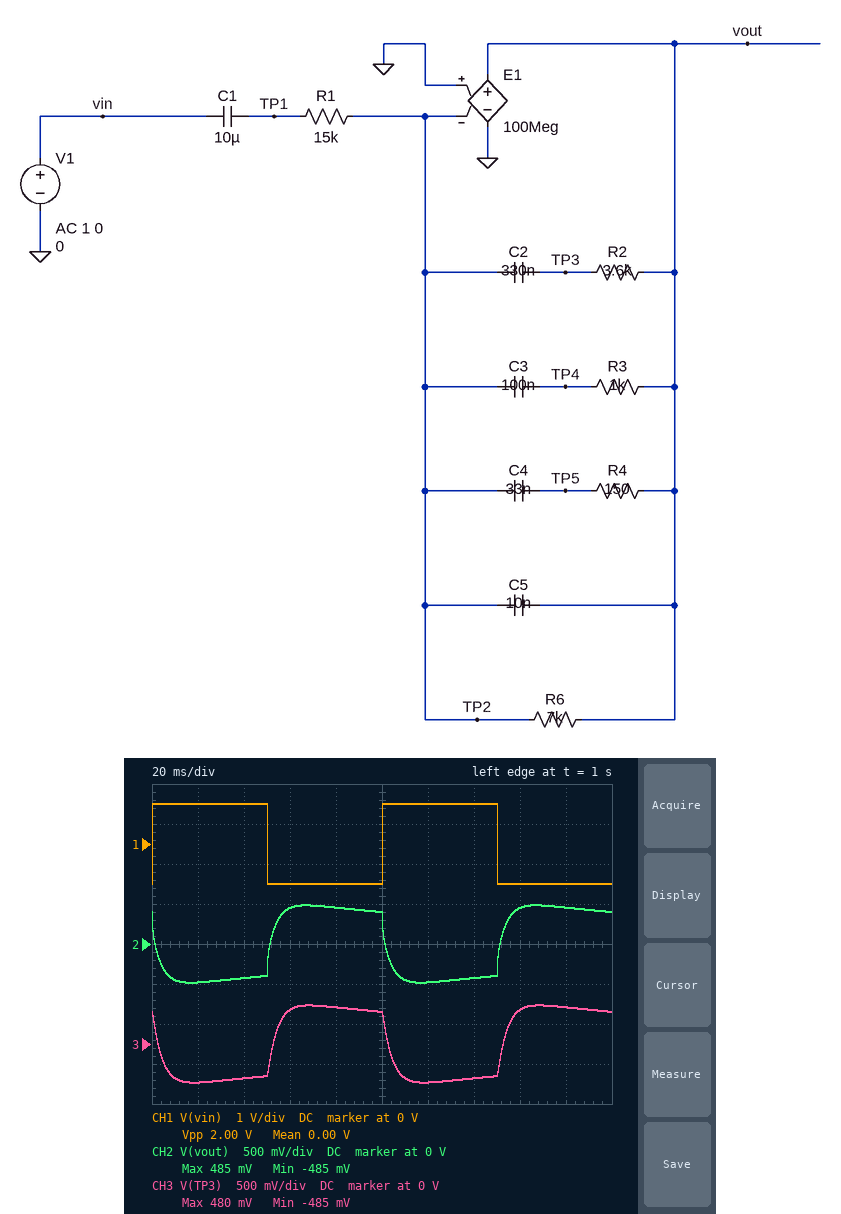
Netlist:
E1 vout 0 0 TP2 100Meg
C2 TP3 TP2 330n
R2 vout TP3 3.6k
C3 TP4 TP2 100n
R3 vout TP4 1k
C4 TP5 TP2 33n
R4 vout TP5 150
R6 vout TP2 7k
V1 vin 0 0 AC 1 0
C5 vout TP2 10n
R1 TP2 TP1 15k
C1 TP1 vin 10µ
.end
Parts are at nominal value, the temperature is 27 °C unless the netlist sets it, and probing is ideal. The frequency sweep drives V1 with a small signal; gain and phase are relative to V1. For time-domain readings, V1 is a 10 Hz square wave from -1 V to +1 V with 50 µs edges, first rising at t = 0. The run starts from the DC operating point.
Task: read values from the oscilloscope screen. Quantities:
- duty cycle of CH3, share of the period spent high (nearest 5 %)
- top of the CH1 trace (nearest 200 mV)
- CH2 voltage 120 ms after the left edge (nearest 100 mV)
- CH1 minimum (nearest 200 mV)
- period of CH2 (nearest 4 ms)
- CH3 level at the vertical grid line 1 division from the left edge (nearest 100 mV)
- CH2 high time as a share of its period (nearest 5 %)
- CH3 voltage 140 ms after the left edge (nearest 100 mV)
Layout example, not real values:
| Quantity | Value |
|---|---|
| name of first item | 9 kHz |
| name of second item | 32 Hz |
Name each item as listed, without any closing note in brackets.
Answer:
| Quantity | Value |
|---|---|
| duty cycle of CH3, share of the period spent high | 50 % |
| top of the CH1 trace | 1.0 V |
| CH2 voltage 120 ms after the left edge | -500 mV |
| CH1 minimum | -1.0 V |
| period of CH2 | 100 ms |
| CH3 level at the vertical grid line 1 division from the left edge | -500 mV |
| CH2 high time as a share of its period | 50 % |
| CH3 voltage 140 ms after the left edge | -400 mV |
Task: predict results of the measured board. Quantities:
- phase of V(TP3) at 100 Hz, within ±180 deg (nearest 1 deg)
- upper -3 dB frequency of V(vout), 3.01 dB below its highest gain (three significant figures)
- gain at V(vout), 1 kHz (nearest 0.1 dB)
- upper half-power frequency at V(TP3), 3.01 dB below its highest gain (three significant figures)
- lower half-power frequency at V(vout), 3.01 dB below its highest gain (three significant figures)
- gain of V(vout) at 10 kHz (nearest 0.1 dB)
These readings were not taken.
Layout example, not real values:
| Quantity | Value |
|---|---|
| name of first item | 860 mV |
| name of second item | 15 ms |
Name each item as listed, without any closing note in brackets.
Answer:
| Quantity | Value |
|---|---|
| phase of V(TP3) at 100 Hz, within ±180 deg | 102 deg |
| upper -3 dB frequency of V(vout), 3.01 dB below its highest gain | 43.0 Hz |
| gain at V(vout), 1 kHz | -23.8 dB |
| upper half-power frequency at V(TP3), 3.01 dB below its highest gain | 39.4 Hz |
| lower half-power frequency at V(vout), 3.01 dB below its highest gain | 1.01 Hz |
| gain of V(vout) at 10 kHz | -34.0 dB |
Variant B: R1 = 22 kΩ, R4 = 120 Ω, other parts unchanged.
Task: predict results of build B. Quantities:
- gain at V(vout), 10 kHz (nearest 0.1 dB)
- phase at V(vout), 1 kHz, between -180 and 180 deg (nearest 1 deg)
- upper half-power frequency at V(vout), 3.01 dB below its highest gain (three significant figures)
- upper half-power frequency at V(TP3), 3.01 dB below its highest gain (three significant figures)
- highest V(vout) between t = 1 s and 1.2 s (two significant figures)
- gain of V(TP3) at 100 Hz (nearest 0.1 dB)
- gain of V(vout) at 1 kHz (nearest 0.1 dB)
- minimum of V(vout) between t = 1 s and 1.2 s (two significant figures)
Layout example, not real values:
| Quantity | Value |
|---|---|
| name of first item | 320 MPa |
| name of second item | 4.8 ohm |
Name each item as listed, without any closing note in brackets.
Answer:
| Quantity | Value |
|---|---|
| gain at V(vout), 10 kHz | -37.3 dB |
| phase at V(vout), 1 kHz, between -180 and 180 deg | 133 deg |
| upper half-power frequency at V(vout), 3.01 dB below its highest gain | 42.3 Hz |
| upper half-power frequency at V(TP3), 3.01 dB below its highest gain | 38.8 Hz |
| highest V(vout) between t = 1 s and 1.2 s | 320 mV |
| gain of V(TP3) at 100 Hz | -19.2 dB |
| gain of V(vout) at 1 kHz | -27.1 dB |
| minimum of V(vout) between t = 1 s and 1.2 s | -330 mV |
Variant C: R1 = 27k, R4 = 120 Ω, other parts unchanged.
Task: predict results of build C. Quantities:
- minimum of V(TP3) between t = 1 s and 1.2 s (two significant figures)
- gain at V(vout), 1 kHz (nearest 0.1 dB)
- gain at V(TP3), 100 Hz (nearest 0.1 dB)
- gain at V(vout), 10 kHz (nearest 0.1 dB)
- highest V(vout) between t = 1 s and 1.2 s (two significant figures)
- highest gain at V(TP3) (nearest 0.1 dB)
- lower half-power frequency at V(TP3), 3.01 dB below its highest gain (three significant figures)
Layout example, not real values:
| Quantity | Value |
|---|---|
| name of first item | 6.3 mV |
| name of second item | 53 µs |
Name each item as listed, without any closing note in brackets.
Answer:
| Quantity | Value |
|---|---|
| minimum of V(TP3) between t = 1 s and 1.2 s | -270 mV |
| gain at V(vout), 1 kHz | -28.9 dB |
| gain at V(TP3), 100 Hz | -21.0 dB |
| gain at V(vout), 10 kHz | -39.1 dB |
| highest V(vout) between t = 1 s and 1.2 s | 260 mV |
| highest gain at V(TP3) | -11.9 dB |
| lower half-power frequency at V(TP3), 3.01 dB below its highest gain | 572 mHz |
